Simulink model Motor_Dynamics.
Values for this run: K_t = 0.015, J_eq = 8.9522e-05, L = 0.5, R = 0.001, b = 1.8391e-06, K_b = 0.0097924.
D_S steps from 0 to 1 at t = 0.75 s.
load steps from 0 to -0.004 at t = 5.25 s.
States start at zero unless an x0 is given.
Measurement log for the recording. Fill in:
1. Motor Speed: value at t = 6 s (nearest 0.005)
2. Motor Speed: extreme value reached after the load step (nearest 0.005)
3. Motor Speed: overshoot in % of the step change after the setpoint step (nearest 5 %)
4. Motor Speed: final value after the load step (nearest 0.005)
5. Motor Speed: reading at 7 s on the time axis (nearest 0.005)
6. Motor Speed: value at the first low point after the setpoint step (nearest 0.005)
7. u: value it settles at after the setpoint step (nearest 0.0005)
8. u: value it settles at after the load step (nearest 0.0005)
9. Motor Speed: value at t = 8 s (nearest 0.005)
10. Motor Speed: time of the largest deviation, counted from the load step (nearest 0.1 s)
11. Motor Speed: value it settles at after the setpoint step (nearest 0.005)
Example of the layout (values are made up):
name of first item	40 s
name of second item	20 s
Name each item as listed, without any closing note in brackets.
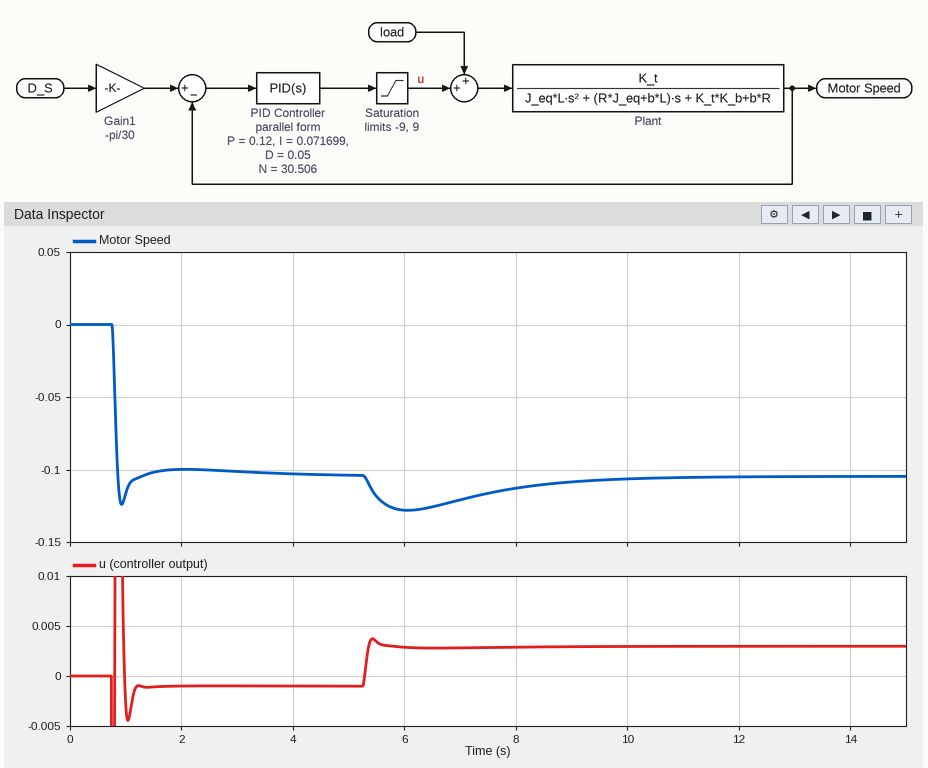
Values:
Motor Speed: value at t = 6 s	-0.130
Motor Speed: extreme value reached after the load step	-0.130
Motor Speed: overshoot in % of the step change after the setpoint step	20 %
Motor Speed: final value after the load step	-0.105
Motor Speed: reading at 7 s on the time axis	-0.120
Motor Speed: value at the first low point after the setpoint step	-0.125
u: value it settles at after the setpoint step	-0.0010
u: value it settles at after the load step	0.0030
Motor Speed: value at t = 8 s	-0.115
Motor Speed: time of the largest deviation, counted from the load step	0.8 s
Motor Speed: value it settles at after the setpoint step	-0.105
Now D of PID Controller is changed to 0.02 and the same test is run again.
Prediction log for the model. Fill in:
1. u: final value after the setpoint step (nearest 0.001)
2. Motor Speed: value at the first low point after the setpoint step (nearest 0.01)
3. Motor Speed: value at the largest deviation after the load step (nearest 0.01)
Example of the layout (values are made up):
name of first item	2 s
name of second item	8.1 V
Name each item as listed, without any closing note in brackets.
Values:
u: final value after the setpoint step	-0.001
Motor Speed: value at the first low point after the setpoint step	-0.14
Motor Speed: value at the largest deviation after the load step	-0.14
